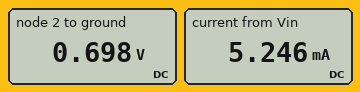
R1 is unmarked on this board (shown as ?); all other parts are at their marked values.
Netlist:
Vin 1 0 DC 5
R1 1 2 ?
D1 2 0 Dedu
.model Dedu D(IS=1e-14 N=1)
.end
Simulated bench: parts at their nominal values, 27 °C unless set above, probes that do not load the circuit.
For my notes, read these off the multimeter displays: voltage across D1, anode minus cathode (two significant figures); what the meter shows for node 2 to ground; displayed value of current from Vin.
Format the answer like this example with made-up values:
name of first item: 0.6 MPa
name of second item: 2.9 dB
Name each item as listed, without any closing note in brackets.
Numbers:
voltage across D1, anode minus cathode: 700 mV
what the meter shows for node 2 to ground: 0.698 V
displayed value of current from Vin: 5.246 mA
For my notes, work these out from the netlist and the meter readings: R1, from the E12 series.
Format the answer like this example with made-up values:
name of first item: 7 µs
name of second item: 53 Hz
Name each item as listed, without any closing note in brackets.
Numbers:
R1, from the E12 series: 820 Ω
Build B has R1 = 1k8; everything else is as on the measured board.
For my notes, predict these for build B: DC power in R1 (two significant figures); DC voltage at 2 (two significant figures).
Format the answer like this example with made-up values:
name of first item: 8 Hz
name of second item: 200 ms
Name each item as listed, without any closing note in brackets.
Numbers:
DC power in R1: 10 mW
DC voltage at 2: 680 mV
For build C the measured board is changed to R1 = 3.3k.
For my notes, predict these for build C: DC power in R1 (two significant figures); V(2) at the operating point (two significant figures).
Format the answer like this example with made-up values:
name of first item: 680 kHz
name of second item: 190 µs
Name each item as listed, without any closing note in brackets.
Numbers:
DC power in R1: 5.7 mW
V(2) at the operating point: 660 mV
